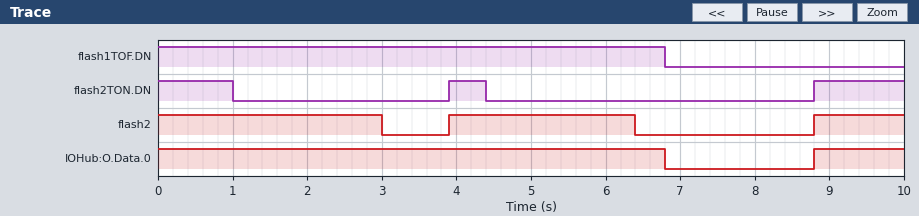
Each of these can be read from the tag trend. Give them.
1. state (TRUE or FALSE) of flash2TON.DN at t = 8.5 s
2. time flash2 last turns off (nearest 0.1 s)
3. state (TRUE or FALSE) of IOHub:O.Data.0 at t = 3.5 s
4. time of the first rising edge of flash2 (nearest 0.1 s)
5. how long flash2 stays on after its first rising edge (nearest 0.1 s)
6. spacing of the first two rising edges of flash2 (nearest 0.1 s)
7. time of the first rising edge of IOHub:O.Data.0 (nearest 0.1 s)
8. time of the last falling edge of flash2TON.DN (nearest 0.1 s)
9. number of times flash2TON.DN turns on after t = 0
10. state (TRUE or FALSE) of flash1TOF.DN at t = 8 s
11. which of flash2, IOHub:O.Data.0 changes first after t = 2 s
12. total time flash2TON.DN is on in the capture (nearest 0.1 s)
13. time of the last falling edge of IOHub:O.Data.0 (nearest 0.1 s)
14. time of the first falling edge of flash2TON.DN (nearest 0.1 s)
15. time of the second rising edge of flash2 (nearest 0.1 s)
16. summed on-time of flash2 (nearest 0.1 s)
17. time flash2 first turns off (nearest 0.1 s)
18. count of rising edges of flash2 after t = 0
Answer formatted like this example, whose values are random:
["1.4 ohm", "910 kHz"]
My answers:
["FALSE", "6.4 s", "TRUE", "3.9 s", "2.5 s", "4.9 s", "8.8 s", "4.4 s", "2", "FALSE", "flash2", "2.7 s", "6.8 s", "1.0 s", "8.8 s", "6.7 s", "3.0 s", "2"]
